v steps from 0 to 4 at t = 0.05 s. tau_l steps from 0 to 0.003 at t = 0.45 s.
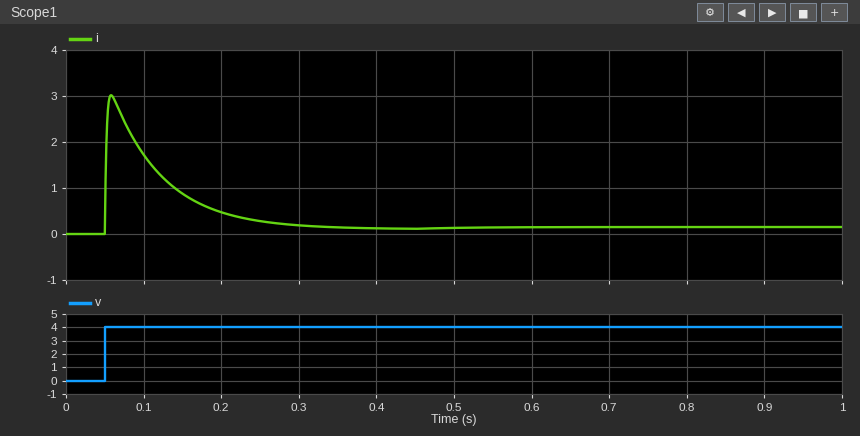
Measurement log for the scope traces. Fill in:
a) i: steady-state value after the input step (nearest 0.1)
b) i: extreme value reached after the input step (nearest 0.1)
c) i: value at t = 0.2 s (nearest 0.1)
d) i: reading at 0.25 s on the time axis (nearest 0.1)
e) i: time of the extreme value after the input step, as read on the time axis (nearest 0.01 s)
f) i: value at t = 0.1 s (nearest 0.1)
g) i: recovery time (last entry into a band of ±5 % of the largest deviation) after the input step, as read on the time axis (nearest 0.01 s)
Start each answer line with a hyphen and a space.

- 0.1
- 3.0
- 0.5
- 0.3
- 0.06 s
- 1.7
- 0.26 s
